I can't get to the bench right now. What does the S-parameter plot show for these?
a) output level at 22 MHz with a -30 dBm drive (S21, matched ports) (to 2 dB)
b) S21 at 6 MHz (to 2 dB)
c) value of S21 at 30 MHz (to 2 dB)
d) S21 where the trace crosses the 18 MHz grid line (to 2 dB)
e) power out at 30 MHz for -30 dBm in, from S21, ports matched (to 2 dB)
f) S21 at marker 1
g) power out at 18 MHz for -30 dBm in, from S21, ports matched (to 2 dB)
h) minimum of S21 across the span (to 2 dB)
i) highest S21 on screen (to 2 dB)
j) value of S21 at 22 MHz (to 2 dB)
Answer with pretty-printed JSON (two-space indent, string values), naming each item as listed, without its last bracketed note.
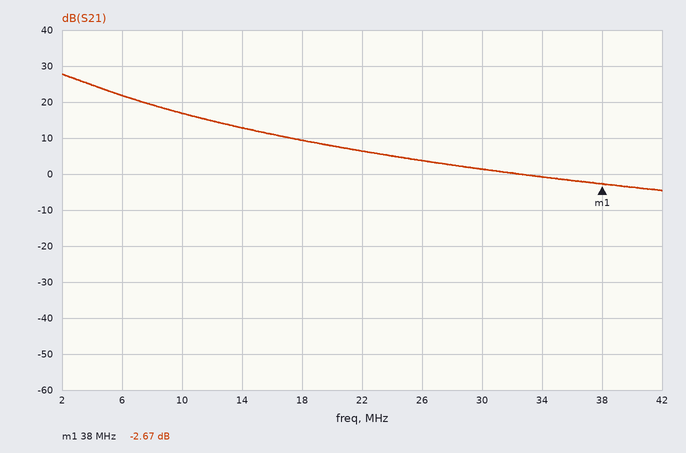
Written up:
{
  "output level at 22 MHz with a -30 dBm drive (S21, matched ports)": "-24 dBm",
  "S21 at 6 MHz": "22 dB",
  "value of S21 at 30 MHz": "2 dB",
  "S21 where the trace crosses the 18 MHz grid line": "10 dB",
  "power out at 30 MHz for -30 dBm in, from S21, ports matched": "-28 dBm",
  "S21 at marker 1": "-2.67 dB",
  "power out at 18 MHz for -30 dBm in, from S21, ports matched": "-20 dBm",
  "minimum of S21 across the span": "-4 dB",
  "highest S21 on screen": "28 dB",
  "value of S21 at 22 MHz": "6 dB"
}
